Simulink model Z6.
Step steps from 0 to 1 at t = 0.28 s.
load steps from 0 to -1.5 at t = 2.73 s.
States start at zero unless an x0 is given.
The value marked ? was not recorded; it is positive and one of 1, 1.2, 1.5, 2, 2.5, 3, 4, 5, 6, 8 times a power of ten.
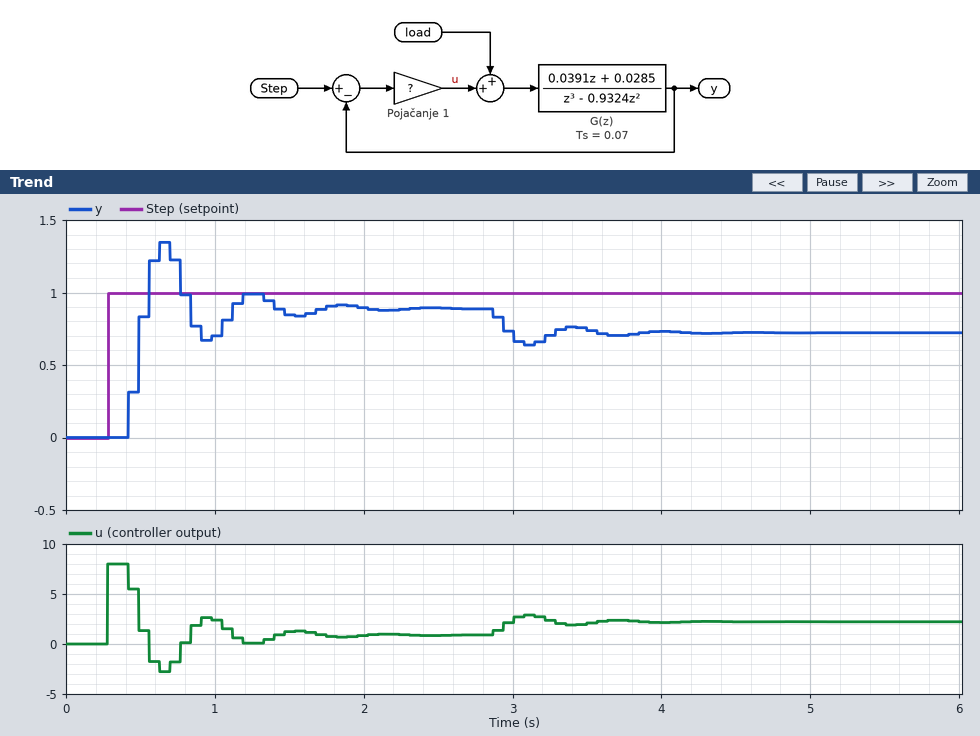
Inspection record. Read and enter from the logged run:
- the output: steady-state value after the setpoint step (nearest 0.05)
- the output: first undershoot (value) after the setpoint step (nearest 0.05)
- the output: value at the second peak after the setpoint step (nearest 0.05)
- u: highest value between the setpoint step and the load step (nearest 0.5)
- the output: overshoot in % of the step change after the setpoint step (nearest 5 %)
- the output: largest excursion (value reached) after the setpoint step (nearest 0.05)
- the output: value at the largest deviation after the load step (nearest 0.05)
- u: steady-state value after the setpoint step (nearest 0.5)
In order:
0.90
0.65
1.00
8.0
50 %
1.35
0.65
1.0
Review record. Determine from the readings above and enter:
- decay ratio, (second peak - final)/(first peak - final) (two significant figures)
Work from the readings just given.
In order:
0.22
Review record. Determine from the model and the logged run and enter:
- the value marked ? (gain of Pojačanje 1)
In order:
8
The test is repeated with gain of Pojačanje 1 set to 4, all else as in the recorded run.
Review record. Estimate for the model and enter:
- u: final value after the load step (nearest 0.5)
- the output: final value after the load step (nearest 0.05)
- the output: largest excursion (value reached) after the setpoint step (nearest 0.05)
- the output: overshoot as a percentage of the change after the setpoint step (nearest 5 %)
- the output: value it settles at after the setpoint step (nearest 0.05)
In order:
2.0
0.50
0.85
10 %
0.80
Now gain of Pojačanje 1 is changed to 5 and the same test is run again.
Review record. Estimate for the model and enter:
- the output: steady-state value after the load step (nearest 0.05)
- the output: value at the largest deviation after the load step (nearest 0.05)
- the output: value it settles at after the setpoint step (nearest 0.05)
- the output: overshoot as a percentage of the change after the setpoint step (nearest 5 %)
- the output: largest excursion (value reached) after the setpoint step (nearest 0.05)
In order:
0.60
0.55
0.85
20 %
1.00
